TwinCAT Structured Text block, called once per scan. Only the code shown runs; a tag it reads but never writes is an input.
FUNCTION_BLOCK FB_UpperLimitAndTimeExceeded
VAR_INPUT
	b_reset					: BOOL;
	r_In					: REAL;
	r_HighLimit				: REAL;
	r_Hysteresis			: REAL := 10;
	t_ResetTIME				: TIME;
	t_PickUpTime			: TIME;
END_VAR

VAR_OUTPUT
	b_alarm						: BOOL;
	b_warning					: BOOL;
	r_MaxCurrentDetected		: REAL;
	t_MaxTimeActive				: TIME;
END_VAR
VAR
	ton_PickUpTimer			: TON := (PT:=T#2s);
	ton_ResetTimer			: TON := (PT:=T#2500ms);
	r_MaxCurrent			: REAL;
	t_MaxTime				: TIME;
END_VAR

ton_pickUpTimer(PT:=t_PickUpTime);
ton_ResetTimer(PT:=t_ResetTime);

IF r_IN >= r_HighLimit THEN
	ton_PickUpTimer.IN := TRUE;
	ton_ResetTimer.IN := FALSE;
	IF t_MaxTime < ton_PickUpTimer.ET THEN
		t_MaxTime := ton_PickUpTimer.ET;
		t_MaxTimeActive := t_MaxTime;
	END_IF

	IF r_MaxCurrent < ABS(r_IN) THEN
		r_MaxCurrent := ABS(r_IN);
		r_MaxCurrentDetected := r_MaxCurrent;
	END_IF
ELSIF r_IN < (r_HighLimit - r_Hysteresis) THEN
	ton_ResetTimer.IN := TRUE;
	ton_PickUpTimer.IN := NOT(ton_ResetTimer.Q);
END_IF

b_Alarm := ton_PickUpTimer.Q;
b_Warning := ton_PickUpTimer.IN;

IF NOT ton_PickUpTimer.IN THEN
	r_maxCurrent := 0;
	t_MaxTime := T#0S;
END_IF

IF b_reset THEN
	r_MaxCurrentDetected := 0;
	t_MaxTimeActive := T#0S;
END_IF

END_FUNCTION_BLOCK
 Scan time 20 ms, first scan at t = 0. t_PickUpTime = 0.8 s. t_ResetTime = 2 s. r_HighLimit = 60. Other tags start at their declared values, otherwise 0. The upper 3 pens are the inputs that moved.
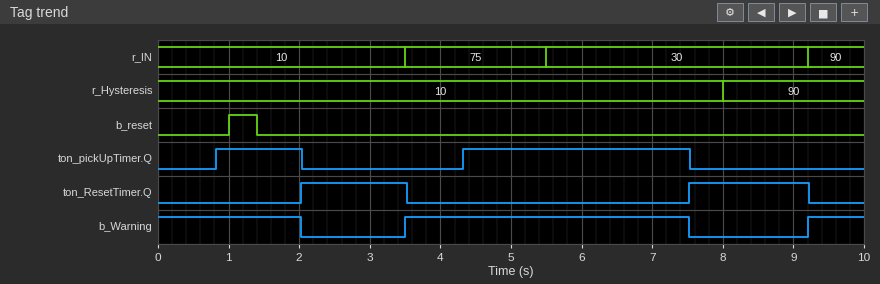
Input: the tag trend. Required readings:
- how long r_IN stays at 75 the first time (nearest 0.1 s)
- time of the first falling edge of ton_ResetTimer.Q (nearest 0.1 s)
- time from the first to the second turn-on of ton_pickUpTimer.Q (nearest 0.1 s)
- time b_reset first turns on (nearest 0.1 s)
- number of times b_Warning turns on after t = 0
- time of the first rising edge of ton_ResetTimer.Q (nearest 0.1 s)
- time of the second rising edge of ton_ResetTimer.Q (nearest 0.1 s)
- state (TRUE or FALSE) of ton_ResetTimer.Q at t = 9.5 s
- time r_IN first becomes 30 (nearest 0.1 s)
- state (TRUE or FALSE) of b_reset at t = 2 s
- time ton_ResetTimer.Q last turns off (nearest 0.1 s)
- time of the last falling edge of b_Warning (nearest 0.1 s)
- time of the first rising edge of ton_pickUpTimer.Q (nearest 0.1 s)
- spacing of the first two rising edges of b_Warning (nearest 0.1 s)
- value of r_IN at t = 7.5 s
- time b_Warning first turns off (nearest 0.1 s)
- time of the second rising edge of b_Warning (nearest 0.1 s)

2.0 s
3.5 s
3.5 s
1.0 s
2
2.0 s
7.5 s
FALSE
5.5 s
FALSE
9.2 s
7.5 s
0.8 s
5.7 s
30
2.0 s
9.2 s
